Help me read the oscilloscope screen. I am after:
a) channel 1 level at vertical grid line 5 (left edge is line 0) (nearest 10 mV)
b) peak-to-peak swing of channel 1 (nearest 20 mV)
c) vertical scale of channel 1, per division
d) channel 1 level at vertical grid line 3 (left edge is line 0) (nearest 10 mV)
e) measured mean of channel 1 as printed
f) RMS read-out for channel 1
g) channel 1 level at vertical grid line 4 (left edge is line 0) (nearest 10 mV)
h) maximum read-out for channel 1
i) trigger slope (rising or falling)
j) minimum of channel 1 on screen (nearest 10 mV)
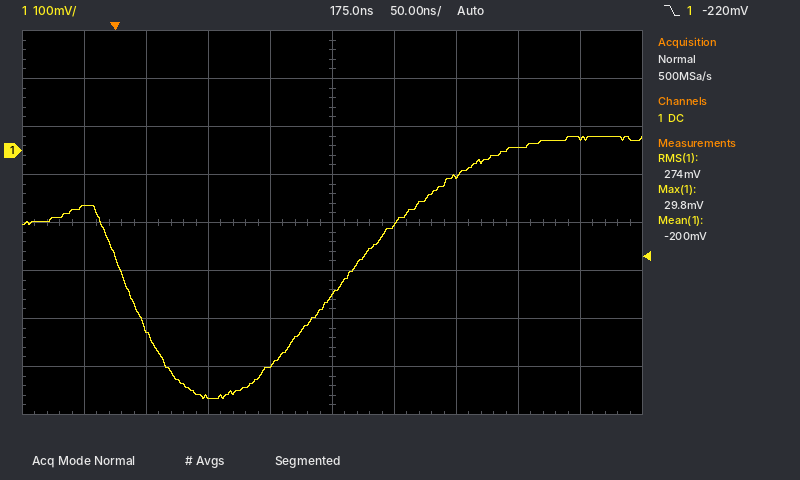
-300 mV
540 mV
100 mV
-510 mV
-200 mV
274 mV
-450 mV
29.8 mV
falling
-520 mV
